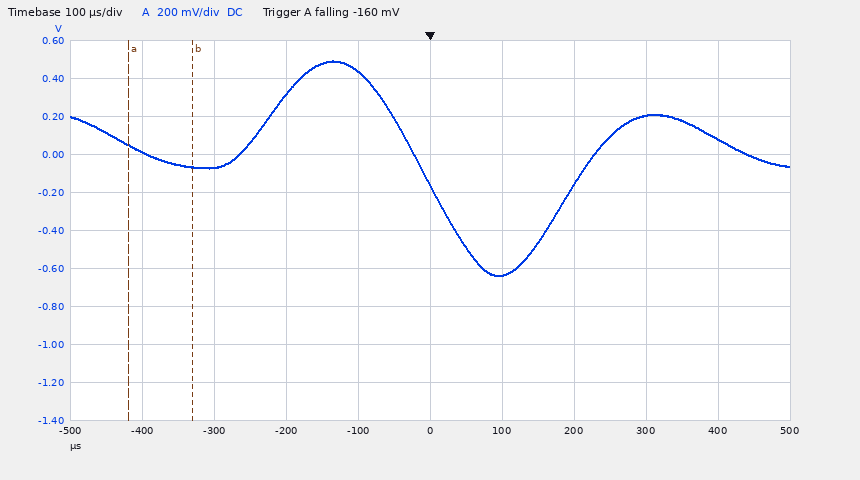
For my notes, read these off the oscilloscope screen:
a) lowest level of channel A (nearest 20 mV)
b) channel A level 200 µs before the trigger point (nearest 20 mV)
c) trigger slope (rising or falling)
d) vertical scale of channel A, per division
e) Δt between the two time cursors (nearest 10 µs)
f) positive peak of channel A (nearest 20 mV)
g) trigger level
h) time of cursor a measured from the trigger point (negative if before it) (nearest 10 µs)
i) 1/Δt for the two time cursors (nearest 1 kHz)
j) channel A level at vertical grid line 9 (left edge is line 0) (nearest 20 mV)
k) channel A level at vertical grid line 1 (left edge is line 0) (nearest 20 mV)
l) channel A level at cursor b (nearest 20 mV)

-640 mV
320 mV
falling
200 mV
90 µs
500 mV
-160 mV
-420 µs
11 kHz
80 mV
20 mV
-60 mV
